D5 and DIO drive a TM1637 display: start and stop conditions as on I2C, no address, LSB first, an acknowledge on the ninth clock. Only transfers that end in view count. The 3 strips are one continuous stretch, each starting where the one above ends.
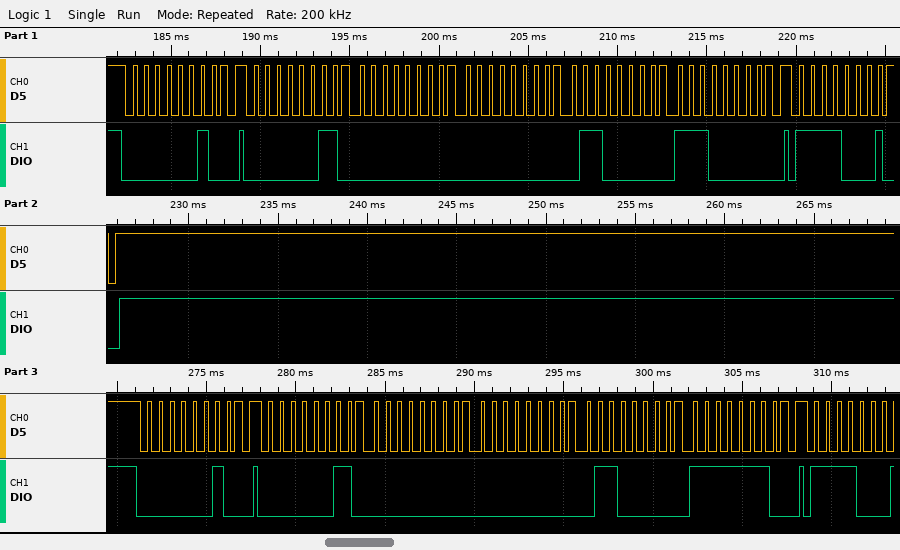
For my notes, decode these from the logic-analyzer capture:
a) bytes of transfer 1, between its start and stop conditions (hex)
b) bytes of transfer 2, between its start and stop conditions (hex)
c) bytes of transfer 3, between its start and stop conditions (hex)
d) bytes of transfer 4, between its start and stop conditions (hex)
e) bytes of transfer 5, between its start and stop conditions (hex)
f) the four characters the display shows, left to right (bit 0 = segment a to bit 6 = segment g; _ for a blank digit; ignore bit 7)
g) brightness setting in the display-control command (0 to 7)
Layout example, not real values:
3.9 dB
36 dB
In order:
40
C0 00 00 06 07
8F
40
C0 00 00 06 7F
__18
7
